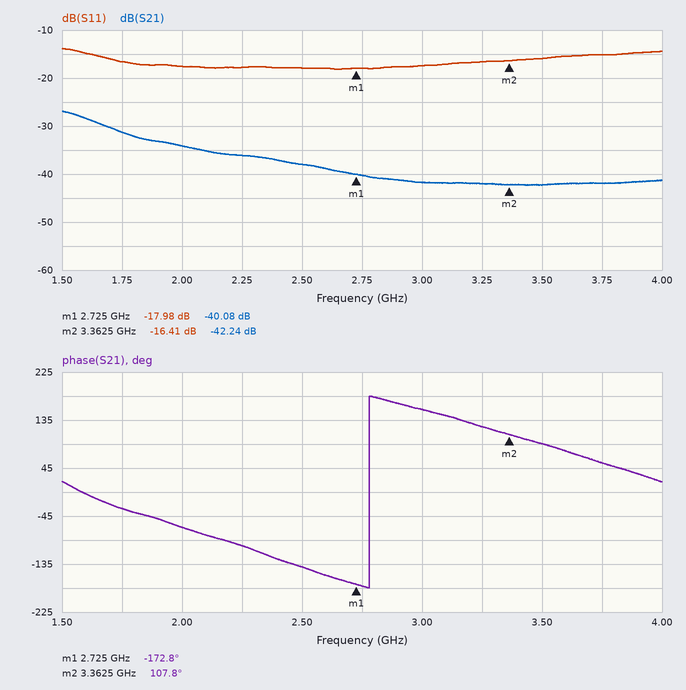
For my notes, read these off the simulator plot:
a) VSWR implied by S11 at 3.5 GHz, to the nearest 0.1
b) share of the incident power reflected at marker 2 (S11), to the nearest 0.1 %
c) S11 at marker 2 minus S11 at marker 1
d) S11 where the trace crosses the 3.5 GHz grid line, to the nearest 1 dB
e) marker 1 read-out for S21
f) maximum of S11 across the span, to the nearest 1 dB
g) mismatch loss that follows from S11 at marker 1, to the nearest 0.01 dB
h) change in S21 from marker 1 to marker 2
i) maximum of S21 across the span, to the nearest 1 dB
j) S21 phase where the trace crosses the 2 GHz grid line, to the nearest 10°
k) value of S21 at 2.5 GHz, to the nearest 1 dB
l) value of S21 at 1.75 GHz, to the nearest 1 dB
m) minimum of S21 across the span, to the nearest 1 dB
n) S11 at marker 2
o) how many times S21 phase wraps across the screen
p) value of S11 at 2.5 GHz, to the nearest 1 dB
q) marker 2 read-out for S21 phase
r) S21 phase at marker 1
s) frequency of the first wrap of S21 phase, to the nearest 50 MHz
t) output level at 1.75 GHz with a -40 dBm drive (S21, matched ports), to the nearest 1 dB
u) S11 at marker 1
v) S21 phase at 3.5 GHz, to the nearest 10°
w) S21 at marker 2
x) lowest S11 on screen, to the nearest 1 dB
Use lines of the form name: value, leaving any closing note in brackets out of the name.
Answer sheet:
VSWR implied by S11 at 3.5 GHz, to the nearest 0.1: 1.4
share of the incident power reflected at marker 2 (S11), to the nearest 0.1 %: 2.3 %
S11 at marker 2 minus S11 at marker 1: 1.57 dB
S11 where the trace crosses the 3.5 GHz grid line, to the nearest 1 dB: -16 dB
marker 1 read-out for S21: -40.08 dB
maximum of S11 across the span, to the nearest 1 dB: -14 dB
mismatch loss that follows from S11 at marker 1, to the nearest 0.01 dB: 0.07 dB
change in S21 from marker 1 to marker 2: -2.16 dB
maximum of S21 across the span, to the nearest 1 dB: -27 dB
S21 phase where the trace crosses the 2 GHz grid line, to the nearest 10°: -70°
value of S21 at 2.5 GHz, to the nearest 1 dB: -38 dB
value of S21 at 1.75 GHz, to the nearest 1 dB: -31 dB
minimum of S21 across the span, to the nearest 1 dB: -42 dB
S11 at marker 2: -16.41 dB
how many times S21 phase wraps across the screen: 1
value of S11 at 2.5 GHz, to the nearest 1 dB: -18 dB
marker 2 read-out for S21 phase: 107.8°
S21 phase at marker 1: -172.8°
frequency of the first wrap of S21 phase, to the nearest 50 MHz: 2.80 GHz
output level at 1.75 GHz with a -40 dBm drive (S21, matched ports), to the nearest 1 dB: -71 dBm
S11 at marker 1: -17.98 dB
S21 phase at 3.5 GHz, to the nearest 10°: 90°
S21 at marker 2: -42.24 dB
lowest S11 on screen, to the nearest 1 dB: -18 dB
